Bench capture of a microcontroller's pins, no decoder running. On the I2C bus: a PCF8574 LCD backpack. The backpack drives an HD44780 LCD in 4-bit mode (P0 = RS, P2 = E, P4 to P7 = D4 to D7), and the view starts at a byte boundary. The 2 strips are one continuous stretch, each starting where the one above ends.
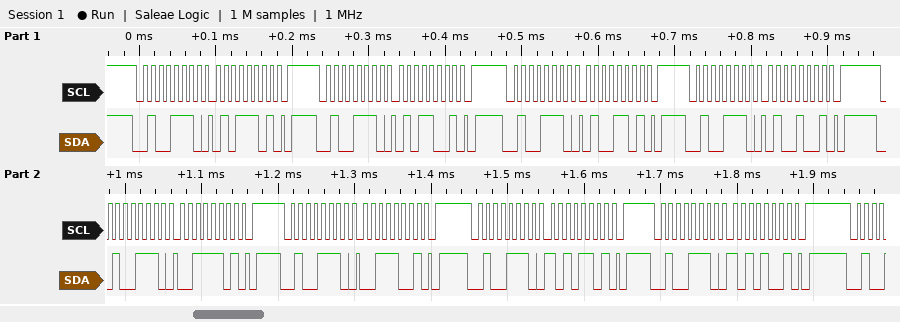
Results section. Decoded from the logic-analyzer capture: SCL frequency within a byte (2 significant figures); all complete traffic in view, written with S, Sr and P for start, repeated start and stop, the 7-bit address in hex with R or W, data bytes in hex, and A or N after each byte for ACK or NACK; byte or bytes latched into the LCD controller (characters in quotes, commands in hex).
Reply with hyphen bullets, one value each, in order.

- 100 kHz
- S 27W A 5D A P S 27W A 59 A P S 27W A 4D A P S 27W A 49 A P S 27W A 3D A P S 27W A 39 A P S 27W A AD A P S 27W A A9 A P
- 'T' ':'
